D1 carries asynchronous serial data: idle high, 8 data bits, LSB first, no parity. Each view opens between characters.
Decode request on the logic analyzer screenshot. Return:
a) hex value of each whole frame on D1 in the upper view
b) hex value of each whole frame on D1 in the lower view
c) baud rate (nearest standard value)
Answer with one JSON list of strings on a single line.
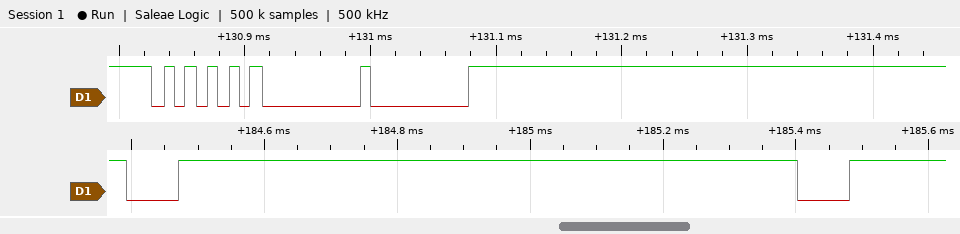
["55, 00, 00", "00, 00", "115200 baud"]
